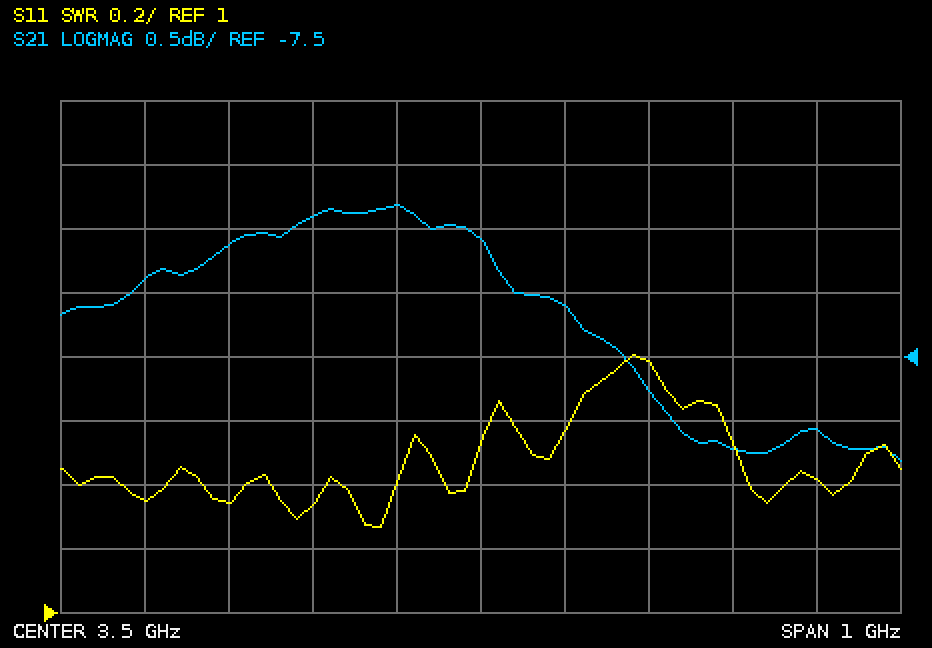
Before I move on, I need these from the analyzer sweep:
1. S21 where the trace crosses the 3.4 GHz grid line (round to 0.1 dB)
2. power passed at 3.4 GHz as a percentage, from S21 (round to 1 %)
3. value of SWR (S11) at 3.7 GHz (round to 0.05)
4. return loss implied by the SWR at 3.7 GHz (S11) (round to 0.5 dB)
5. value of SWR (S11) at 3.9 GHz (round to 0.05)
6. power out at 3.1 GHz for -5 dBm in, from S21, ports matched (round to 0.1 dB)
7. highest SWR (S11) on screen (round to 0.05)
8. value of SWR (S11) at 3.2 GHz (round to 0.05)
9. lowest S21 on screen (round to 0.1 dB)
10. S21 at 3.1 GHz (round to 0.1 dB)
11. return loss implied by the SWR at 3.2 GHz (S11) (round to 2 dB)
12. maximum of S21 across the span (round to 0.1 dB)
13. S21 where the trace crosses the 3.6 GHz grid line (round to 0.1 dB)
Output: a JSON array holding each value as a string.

["-6.3 dB", "23 %", "1.80", "11.0 dB", "1.40", "-11.9 dBm", "1.80", "1.35", "-8.3 dB", "-6.9 dB", "16 dB", "-6.3 dB", "-7.1 dB"]
